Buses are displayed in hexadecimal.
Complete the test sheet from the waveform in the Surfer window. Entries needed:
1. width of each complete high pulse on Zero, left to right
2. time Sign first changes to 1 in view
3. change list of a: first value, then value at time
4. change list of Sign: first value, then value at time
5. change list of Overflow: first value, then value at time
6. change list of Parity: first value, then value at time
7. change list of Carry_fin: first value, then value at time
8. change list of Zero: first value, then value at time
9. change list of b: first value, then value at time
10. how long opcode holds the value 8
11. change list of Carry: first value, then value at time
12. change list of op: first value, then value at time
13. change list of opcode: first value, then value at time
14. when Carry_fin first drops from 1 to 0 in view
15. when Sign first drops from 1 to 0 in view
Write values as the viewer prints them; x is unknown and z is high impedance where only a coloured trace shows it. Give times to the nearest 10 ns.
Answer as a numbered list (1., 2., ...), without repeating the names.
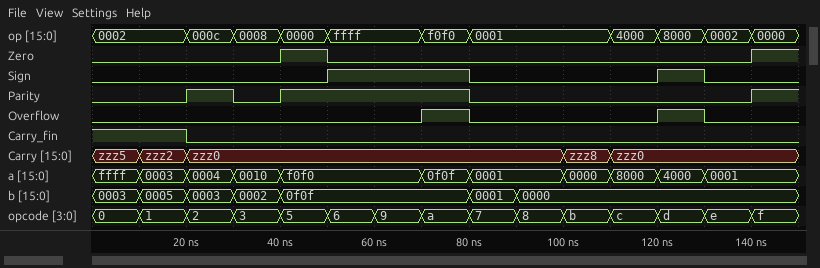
1. 10 ns
2. 50 ns
3. ffff, 0003 at 10 ns, 0004 at 20 ns, 0010 at 30 ns, f0f0 at 40 ns, 0f0f at 70 ns, 0001 at 80 ns, 0000 at 100 ns, 8000 at 110 ns, 4000 at 120 ns, 0001 at 130 ns
4. 0, 1 at 50 ns, 0 at 80 ns, 1 at 120 ns, 0 at 130 ns
5. 0, 1 at 70 ns, 0 at 80 ns, 1 at 120 ns, 0 at 130 ns
6. 0, 1 at 20 ns, 0 at 30 ns, 1 at 40 ns, 0 at 80 ns, 1 at 140 ns
7. 1, 0 at 20 ns
8. 0, 1 at 40 ns, 0 at 50 ns, 1 at 140 ns
9. 0003, 0005 at 10 ns, 0003 at 20 ns, 0002 at 30 ns, 0f0f at 40 ns, 0001 at 80 ns, 0000 at 90 ns
10. 10 ns
11. zzz5, zzz2 at 10 ns, zzz0 at 20 ns, zzz8 at 100 ns, zzz0 at 110 ns
12. 0002, 000c at 20 ns, 0008 at 30 ns, 0000 at 40 ns, ffff at 50 ns, f0f0 at 70 ns, 0001 at 80 ns, 4000 at 110 ns, 8000 at 120 ns, 0002 at 130 ns, 0000 at 140 ns
13. 0, 1 at 10 ns, 2 at 20 ns, 3 at 30 ns, 5 at 40 ns, 6 at 50 ns, 9 at 60 ns, a at 70 ns, 7 at 80 ns, 8 at 90 ns, b at 100 ns, c at 110 ns, d at 120 ns, e at 130 ns, f at 140 ns
14. 20 ns
15. 80 ns
